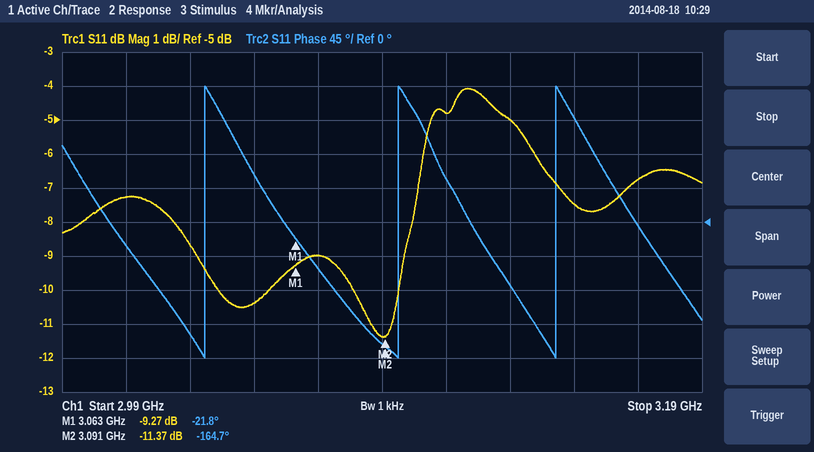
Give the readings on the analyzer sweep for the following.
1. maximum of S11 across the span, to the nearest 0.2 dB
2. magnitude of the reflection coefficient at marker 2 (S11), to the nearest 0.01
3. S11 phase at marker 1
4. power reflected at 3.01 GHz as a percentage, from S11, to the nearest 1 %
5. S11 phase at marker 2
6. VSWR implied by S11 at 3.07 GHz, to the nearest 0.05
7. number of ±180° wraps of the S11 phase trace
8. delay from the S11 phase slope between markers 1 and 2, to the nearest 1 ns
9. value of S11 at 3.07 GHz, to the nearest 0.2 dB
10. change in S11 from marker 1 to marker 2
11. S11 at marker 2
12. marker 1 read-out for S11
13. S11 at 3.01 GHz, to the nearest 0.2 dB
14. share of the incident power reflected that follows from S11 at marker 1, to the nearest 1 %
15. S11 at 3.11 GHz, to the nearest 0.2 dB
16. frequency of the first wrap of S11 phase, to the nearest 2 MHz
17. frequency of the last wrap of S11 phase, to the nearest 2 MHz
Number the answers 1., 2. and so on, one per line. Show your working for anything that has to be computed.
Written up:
1. -4.0 dB
2. 10^(-11.37/20) ≈ 0.27
3. -21.8°
4. 10^(-7.2/10) ≈ 19 %
5. -164.7°
6. |Γ| = 10^(-9/20) = 0.3548; VSWR = (1 + 0.3548)/(1 − 0.3548) ≈ 2.10
7. 3
8. −(-164.7° − (-21.8°))/(360° × 28 MHz) ≈ 14 ns
9. -9.0 dB
10. -11.37 − (-9.27) = -2.10 dB
11. -11.37 dB
12. -9.27 dB
13. -7.2 dB
14. 10^(-9.27/10) ≈ 12 %
15. -4.8 dB
16. 3.034 GHz
17. 3.144 GHz
